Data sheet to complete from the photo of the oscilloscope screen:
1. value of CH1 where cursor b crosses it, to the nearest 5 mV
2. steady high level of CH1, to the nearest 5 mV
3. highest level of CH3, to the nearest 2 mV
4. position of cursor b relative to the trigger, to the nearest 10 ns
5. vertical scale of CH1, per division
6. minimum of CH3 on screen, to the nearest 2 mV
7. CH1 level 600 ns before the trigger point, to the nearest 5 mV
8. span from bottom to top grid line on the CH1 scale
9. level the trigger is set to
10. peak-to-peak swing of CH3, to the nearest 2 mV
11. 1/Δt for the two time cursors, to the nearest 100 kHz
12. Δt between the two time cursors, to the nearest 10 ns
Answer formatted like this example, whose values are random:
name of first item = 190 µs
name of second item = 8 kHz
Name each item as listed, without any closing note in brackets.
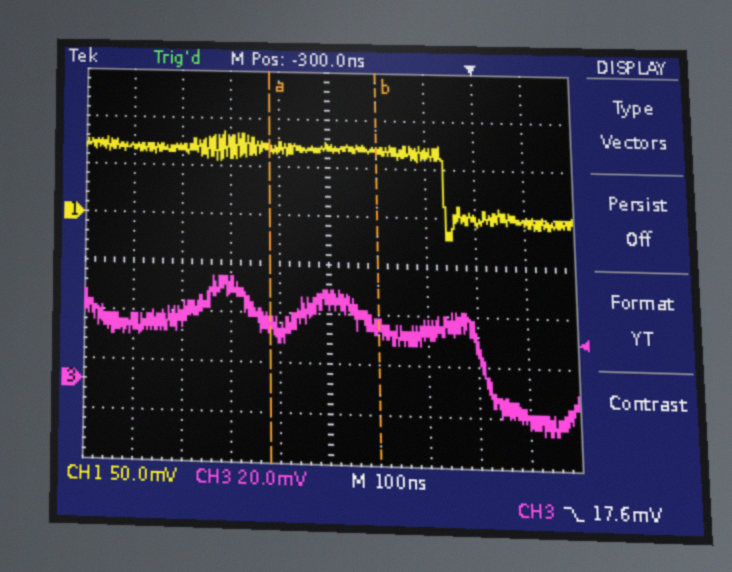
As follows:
value of CH1 where cursor b crosses it, to the nearest 5 mV = 70 mV
steady high level of CH1, to the nearest 5 mV = 70 mV
highest level of CH3, to the nearest 2 mV = 42 mV
position of cursor b relative to the trigger, to the nearest 10 ns = -200 ns
vertical scale of CH1, per division = 50 mV
minimum of CH3 on screen, to the nearest 2 mV = -18 mV
CH1 level 600 ns before the trigger point, to the nearest 5 mV = 70 mV
span from bottom to top grid line on the CH1 scale = 400 mV
level the trigger is set to = 17.6 mV
peak-to-peak swing of CH3, to the nearest 2 mV = 60 mV
1/Δt for the two time cursors, to the nearest 100 kHz = 4.5 MHz
Δt between the two time cursors, to the nearest 10 ns = 220 ns
